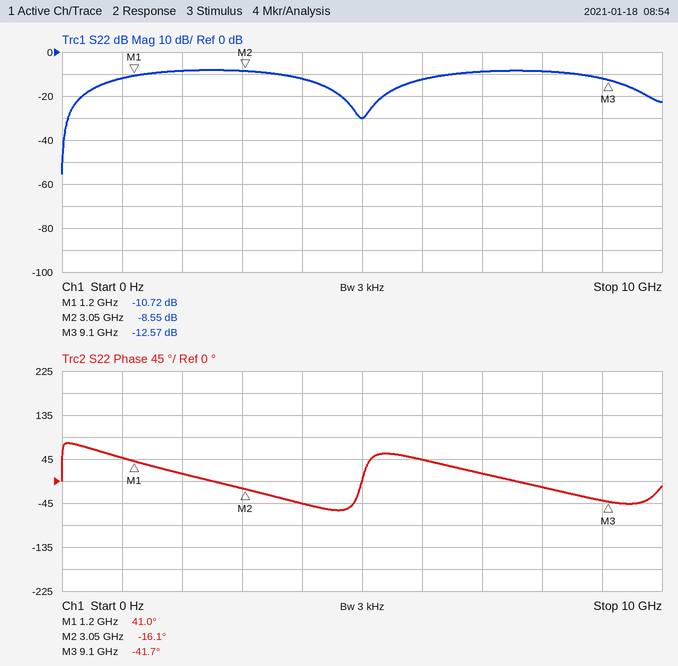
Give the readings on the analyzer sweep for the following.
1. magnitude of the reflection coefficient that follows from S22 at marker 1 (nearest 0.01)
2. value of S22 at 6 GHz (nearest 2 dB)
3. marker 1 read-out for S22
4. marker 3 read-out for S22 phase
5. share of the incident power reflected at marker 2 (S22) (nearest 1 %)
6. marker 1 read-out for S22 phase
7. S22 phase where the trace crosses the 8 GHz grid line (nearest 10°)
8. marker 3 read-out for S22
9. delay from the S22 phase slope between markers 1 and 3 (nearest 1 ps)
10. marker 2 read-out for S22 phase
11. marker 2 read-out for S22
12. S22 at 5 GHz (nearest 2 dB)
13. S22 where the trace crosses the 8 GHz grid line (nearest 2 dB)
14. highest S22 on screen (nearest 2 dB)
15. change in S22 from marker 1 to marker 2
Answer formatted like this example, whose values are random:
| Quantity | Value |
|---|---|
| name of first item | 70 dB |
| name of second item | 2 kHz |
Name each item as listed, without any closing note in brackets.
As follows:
| Quantity | Value |
|---|---|
| magnitude of the reflection coefficient that follows from S22 at marker 1 | 0.29 |
| value of S22 at 6 GHz | -12 dB |
| marker 1 read-out for S22 | -10.72 dB |
| marker 3 read-out for S22 phase | -41.7° |
| share of the incident power reflected at marker 2 (S22) | 14 % |
| marker 1 read-out for S22 phase | 41.0° |
| S22 phase where the trace crosses the 8 GHz grid line | -10° |
| marker 3 read-out for S22 | -12.57 dB |
| delay from the S22 phase slope between markers 1 and 3 | 29 ps |
| marker 2 read-out for S22 phase | -16.1° |
| marker 2 read-out for S22 | -8.55 dB |
| S22 at 5 GHz | -30 dB |
| S22 where the trace crosses the 8 GHz grid line | -8 dB |
| highest S22 on screen | -8 dB |
| change in S22 from marker 1 to marker 2 | 2.17 dB |
